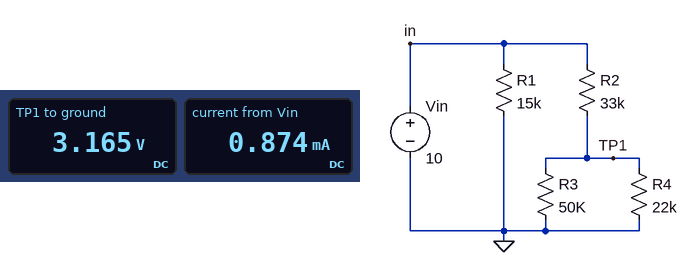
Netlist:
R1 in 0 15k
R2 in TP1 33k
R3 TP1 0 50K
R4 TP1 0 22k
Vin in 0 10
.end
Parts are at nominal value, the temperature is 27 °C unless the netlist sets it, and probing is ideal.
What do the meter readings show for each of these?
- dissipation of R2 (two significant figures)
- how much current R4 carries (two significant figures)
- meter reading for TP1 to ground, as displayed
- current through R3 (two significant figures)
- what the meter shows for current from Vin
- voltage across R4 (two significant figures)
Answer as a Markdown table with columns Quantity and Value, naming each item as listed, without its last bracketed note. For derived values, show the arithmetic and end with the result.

| Quantity | Value |
|---|---|
| dissipation of R2 | (10 V - 3.165 V)^2 / 33 kΩ = 1.4 mW |
| how much current R4 carries | (3.165 V) / 22 kΩ = 140 µA |
| meter reading for TP1 to ground, as displayed | 3.165 V |
| current through R3 | (3.165 V) / 50 kΩ = 63 µA |
| what the meter shows for current from Vin | 0.874 mA |
| voltage across R4 | 3.165 V = 3.2 V |
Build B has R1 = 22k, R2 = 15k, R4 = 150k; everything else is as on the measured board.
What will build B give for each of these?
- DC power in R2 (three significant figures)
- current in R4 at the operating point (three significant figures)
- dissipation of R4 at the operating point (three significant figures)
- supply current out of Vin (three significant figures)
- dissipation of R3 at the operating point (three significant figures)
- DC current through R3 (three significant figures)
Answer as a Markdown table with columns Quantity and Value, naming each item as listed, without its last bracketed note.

| Quantity | Value |
|---|---|
| DC power in R2 | 544 µW |
| current in R4 at the operating point | 47.6 µA |
| dissipation of R4 at the operating point | 340 µW |
| supply current out of Vin | 645 µA |
| dissipation of R3 at the operating point | 1.02 mW |
| DC current through R3 | 143 µA |
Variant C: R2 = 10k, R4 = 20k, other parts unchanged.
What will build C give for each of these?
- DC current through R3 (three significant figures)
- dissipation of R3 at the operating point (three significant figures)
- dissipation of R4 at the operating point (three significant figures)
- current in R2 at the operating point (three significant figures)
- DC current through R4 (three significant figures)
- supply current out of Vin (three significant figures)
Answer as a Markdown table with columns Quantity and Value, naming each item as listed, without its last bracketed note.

| Quantity | Value |
|---|---|
| DC current through R3 | 118 µA |
| dissipation of R3 at the operating point | 692 µW |
| dissipation of R4 at the operating point | 1.73 mW |
| current in R2 at the operating point | 412 µA |
| DC current through R4 | 294 µA |
| supply current out of Vin | 1.08 mA |
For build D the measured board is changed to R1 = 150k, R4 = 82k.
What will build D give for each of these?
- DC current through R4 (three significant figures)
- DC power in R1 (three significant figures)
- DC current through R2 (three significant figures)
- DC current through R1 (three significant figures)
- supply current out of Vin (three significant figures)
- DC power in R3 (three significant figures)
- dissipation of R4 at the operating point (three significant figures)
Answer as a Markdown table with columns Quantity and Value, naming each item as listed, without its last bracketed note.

| Quantity | Value |
|---|---|
| DC current through R4 | 59.1 µA |
| DC power in R1 | 667 µW |
| DC current through R2 | 156 µA |
| DC current through R1 | 66.7 µA |
| supply current out of Vin | 223 µA |
| DC power in R3 | 470 µW |
| dissipation of R4 at the operating point | 287 µW |
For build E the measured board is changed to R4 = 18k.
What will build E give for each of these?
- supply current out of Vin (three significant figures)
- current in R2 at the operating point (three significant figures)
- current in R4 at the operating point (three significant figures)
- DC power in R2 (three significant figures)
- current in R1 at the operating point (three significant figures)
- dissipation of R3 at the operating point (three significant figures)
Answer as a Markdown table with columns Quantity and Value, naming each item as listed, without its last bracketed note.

| Quantity | Value |
|---|---|
| supply current out of Vin | 883 µA |
| current in R2 at the operating point | 216 µA |
| current in R4 at the operating point | 159 µA |
| DC power in R2 | 1.54 mW |
| current in R1 at the operating point | 667 µA |
| dissipation of R3 at the operating point | 164 µW |
